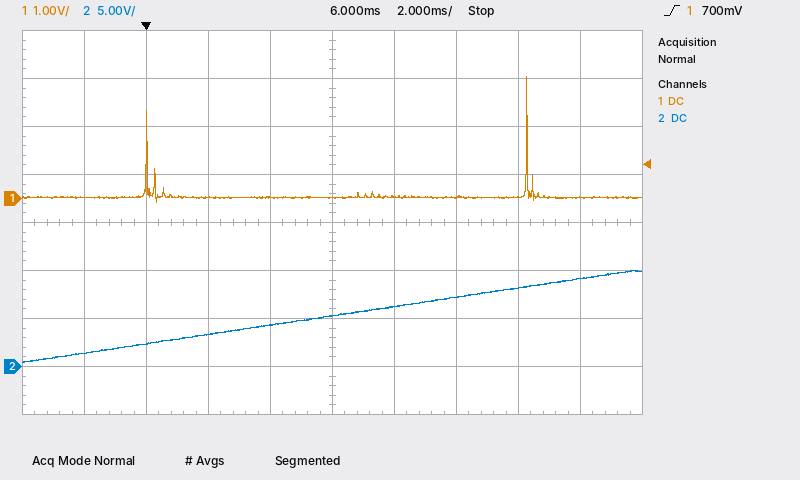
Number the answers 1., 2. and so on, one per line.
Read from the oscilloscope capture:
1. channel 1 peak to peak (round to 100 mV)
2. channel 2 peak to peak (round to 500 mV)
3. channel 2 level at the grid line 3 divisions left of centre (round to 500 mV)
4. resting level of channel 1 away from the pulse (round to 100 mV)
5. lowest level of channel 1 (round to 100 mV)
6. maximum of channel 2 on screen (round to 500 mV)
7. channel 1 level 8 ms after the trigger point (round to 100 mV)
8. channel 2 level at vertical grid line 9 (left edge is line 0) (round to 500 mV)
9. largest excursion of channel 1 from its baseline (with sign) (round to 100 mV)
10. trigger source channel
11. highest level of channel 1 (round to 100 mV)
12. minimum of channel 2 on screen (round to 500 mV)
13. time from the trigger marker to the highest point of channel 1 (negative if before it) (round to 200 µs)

1. 2.6 V
2. 9.5 V
3. 2.5 V
4. 0.0 V
5. -100 mV
6. 10.0 V
7. 0.0 V
8. 9.0 V
9. +2.5 V
10. channel 1
11. 2.5 V
12. 500 mV
13. +12.2 ms
